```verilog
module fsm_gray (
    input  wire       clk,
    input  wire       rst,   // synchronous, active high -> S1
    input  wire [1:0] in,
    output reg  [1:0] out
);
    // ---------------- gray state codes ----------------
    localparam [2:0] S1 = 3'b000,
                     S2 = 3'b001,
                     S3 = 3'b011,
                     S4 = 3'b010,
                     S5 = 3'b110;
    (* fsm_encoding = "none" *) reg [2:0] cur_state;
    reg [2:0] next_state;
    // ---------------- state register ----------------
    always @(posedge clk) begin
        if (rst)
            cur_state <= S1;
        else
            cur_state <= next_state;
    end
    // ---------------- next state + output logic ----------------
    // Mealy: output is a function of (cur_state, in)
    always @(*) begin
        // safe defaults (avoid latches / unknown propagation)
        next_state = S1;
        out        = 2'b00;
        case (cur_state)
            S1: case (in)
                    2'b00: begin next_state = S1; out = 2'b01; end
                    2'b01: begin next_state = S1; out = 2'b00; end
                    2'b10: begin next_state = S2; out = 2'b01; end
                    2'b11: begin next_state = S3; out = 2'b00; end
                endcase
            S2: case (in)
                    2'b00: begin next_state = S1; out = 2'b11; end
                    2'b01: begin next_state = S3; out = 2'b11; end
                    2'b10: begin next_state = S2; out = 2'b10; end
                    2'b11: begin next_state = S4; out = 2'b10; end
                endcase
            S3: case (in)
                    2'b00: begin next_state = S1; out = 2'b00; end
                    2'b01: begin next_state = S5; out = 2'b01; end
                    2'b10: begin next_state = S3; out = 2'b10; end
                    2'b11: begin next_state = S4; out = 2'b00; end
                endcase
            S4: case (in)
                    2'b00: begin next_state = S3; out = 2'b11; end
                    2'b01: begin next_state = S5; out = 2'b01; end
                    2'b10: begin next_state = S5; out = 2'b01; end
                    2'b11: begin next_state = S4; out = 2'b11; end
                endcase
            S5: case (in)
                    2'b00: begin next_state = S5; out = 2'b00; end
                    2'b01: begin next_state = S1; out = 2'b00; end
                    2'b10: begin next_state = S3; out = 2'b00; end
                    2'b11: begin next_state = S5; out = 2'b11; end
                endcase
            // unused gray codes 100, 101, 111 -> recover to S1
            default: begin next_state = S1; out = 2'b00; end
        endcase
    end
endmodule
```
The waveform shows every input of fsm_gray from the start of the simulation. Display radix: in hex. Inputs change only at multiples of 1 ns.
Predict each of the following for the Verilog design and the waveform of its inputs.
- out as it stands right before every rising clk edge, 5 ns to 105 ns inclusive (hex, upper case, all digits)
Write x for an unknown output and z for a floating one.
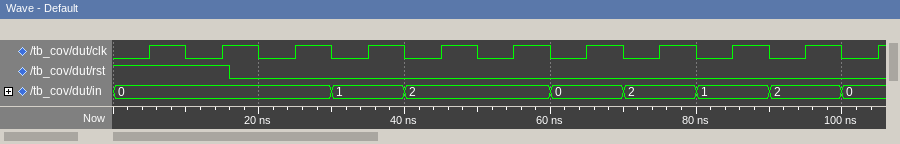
0, 1, 1, 0, 1, 2, 3, 1, 3, 2, 0
